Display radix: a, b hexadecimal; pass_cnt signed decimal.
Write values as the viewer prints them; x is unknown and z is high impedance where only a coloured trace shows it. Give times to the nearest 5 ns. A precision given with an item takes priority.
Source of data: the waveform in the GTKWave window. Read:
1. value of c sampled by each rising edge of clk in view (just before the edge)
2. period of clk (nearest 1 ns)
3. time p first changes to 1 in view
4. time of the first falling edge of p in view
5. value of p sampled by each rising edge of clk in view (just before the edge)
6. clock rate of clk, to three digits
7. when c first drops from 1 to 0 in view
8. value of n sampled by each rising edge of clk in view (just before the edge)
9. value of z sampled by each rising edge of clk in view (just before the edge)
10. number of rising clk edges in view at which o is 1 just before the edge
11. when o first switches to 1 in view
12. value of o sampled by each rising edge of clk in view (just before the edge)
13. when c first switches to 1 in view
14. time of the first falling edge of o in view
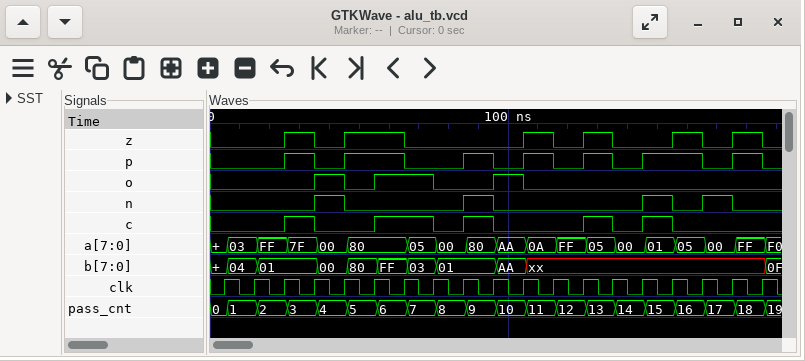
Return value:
0 0 0 1 0 0 1 1 0 1 0 0 0 1 0 1 0 0 0
10 ns
25 ns
35 ns
0 0 0 1 0 1 1 0 0 1 0 1 0 1 0 1 1 0 1
100 MHz
35 ns
0 0 0 0 1 0 0 0 0 1 0 0 0 0 0 1 0 1 0
0 0 0 1 0 1 1 0 0 0 0 1 0 1 0 0 1 0 1
4
35 ns
0 0 0 0 1 0 1 1 0 0 1 0 0 0 0 0 0 0 0
25 ns
45 ns
